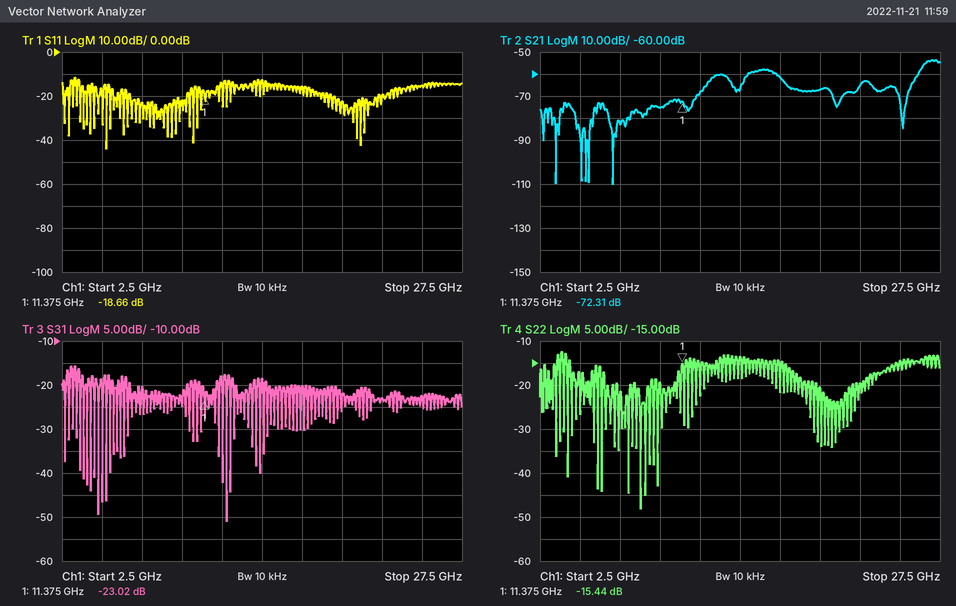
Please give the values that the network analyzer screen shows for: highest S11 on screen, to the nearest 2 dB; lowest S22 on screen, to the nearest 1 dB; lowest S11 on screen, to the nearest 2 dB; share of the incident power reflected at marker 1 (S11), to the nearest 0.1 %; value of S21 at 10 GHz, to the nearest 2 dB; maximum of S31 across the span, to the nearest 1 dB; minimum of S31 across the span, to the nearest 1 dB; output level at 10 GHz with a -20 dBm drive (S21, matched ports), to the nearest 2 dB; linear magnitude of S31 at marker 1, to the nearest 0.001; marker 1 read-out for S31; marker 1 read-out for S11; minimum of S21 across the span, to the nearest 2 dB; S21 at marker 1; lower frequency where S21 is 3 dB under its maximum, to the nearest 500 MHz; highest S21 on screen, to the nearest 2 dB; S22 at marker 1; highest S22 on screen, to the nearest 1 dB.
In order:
-12 dB
-48 dB
-44 dB
1.4 %
-76 dB
-16 dB
-51 dB
-96 dBm
0.071
-23.02 dB
-18.66 dB
-110 dB
-72.31 dB
26.5 GHz
-54 dB
-15.44 dB
-12 dB
